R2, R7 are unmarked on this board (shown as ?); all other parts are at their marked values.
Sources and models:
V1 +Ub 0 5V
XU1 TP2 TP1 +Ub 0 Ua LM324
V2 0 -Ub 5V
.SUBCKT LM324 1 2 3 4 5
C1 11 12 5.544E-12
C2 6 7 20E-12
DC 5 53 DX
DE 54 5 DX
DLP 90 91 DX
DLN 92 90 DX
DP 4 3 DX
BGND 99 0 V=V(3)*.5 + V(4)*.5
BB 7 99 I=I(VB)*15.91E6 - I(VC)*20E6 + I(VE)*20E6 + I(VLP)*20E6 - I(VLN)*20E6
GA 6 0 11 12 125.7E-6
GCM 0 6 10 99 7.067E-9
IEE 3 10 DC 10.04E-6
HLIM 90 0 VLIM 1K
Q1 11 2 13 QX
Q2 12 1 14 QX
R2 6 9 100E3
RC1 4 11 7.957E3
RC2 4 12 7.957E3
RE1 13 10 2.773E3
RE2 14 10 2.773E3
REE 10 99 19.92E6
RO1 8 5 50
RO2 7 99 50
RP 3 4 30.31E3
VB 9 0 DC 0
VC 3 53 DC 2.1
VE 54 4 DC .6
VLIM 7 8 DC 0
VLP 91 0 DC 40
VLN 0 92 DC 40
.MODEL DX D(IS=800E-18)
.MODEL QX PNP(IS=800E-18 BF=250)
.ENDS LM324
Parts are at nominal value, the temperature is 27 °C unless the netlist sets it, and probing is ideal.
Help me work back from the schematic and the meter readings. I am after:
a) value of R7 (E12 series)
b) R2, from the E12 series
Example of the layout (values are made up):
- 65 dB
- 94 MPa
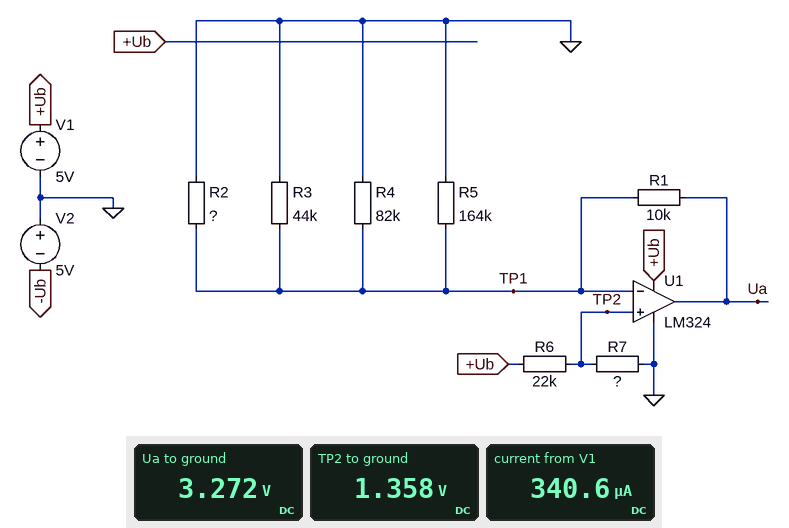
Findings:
- 8.2 kΩ
- 10 kΩ
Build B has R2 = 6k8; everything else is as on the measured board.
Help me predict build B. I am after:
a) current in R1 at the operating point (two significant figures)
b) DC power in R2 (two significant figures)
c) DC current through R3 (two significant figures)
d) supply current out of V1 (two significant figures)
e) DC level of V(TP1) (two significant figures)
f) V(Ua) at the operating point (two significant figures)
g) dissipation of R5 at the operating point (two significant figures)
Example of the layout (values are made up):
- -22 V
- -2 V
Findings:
- 230 µA
- 220 µW
- 28 µA
- 330 µA
- 1.2 V
- 3.5 V
- 9.0 µW
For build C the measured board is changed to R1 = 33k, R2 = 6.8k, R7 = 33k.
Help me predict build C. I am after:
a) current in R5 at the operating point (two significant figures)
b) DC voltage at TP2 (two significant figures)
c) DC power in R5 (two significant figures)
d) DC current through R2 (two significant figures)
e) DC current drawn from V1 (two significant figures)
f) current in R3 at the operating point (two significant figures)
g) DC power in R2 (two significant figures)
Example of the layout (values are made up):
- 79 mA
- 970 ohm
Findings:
- 3.0 µA
- 3.0 V
- 1.4 µW
- 71 µA
- 260 µA
- 11 µA
- 35 µW
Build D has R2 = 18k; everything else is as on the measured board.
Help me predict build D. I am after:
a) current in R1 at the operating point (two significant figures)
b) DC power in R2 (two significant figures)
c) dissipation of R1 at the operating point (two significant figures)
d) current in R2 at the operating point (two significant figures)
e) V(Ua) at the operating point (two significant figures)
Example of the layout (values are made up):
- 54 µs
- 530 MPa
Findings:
- 130 µA
- 100 µW
- 170 µW
- 75 µA
- 2.7 V
